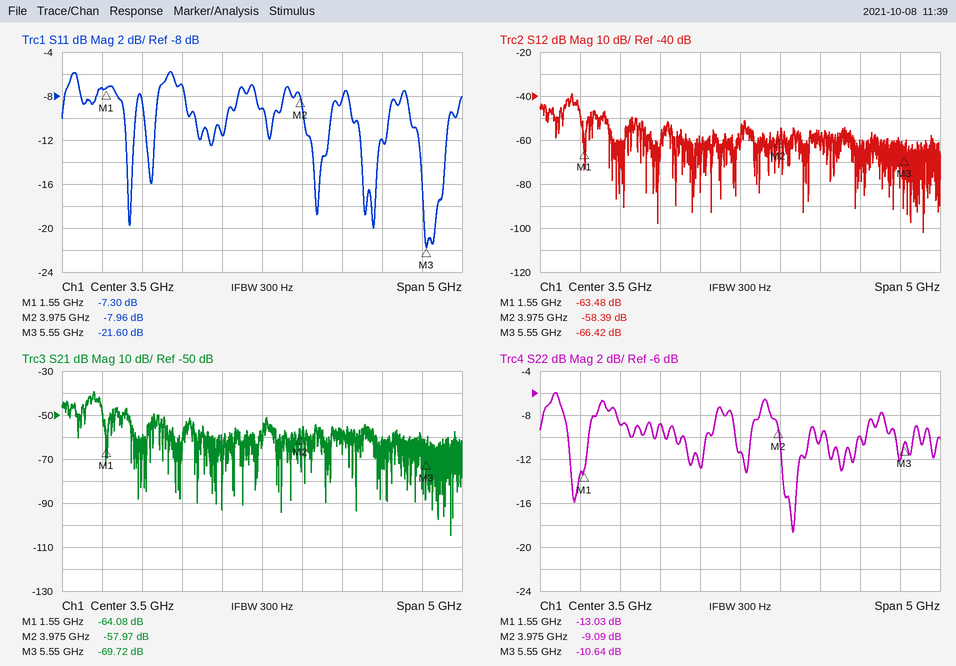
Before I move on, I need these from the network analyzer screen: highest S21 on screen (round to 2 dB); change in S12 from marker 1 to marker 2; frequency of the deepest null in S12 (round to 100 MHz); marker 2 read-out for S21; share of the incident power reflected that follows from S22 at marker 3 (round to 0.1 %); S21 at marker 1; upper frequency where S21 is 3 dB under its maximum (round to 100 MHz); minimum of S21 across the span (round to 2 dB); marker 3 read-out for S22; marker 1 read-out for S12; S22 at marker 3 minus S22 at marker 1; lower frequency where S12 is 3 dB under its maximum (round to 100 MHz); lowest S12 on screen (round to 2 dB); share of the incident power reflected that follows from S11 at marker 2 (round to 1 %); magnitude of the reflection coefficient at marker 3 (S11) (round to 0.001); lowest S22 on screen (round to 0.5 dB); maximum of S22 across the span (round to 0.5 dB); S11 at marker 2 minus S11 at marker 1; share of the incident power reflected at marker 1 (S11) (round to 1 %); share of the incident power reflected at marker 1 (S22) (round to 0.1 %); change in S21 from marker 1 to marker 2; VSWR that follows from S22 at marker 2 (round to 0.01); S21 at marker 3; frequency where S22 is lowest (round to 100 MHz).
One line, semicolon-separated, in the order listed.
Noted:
-40 dB; 5.09 dB; 5.8 GHz; -57.97 dB; 8.6 %; -64.08 dB; 1.4 GHz; -104 dB; -10.64 dB; -63.48 dB; 2.39 dB; 1.4 GHz; -102 dB; 16 %; 0.083; -18.5 dB; -6.0 dB; -0.66 dB; 19 %; 5.0 %; 6.11 dB; 2.08; -69.72 dB; 4.2 GHz
